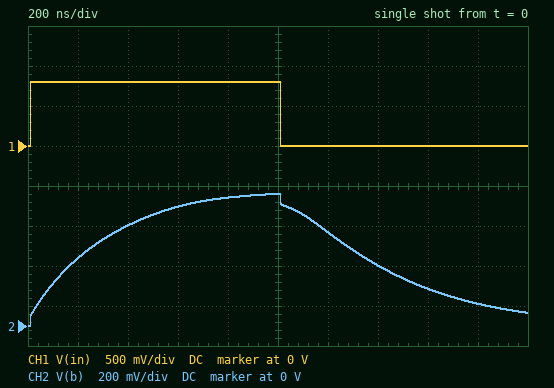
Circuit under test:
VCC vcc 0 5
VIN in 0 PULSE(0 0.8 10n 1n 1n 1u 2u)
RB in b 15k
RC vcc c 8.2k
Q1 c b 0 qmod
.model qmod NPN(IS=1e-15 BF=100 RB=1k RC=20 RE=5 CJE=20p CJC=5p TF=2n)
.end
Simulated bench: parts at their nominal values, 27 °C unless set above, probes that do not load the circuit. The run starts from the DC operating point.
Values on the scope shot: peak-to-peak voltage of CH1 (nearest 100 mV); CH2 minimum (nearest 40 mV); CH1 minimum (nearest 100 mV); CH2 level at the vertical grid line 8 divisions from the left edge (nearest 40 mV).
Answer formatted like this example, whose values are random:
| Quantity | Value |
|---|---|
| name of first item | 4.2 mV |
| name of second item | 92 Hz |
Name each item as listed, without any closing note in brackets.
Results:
| Quantity | Value |
|---|---|
| peak-to-peak voltage of CH1 | 800 mV |
| CH2 minimum | 0 V |
| CH1 minimum | 0 V |
| CH2 level at the vertical grid line 8 divisions from the left edge | 200 mV |
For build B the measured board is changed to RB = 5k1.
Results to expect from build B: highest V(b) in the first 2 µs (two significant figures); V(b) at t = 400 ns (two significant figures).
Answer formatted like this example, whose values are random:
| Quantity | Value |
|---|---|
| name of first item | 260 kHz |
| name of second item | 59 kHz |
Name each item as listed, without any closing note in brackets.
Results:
| Quantity | Value |
|---|---|
| highest V(b) in the first 2 µs | 710 mV |
| V(b) at t = 400 ns | 680 mV |
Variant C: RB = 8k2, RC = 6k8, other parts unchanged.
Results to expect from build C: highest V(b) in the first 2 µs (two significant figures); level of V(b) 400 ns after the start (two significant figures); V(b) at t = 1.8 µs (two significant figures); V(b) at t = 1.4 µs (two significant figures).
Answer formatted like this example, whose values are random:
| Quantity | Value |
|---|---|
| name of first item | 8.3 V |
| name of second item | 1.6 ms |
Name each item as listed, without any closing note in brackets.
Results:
| Quantity | Value |
|---|---|
| highest V(b) in the first 2 µs | 700 mV |
| level of V(b) 400 ns after the start | 630 mV |
| V(b) at t = 1.8 µs | 31 mV |
| V(b) at t = 1.4 µs | 190 mV |
